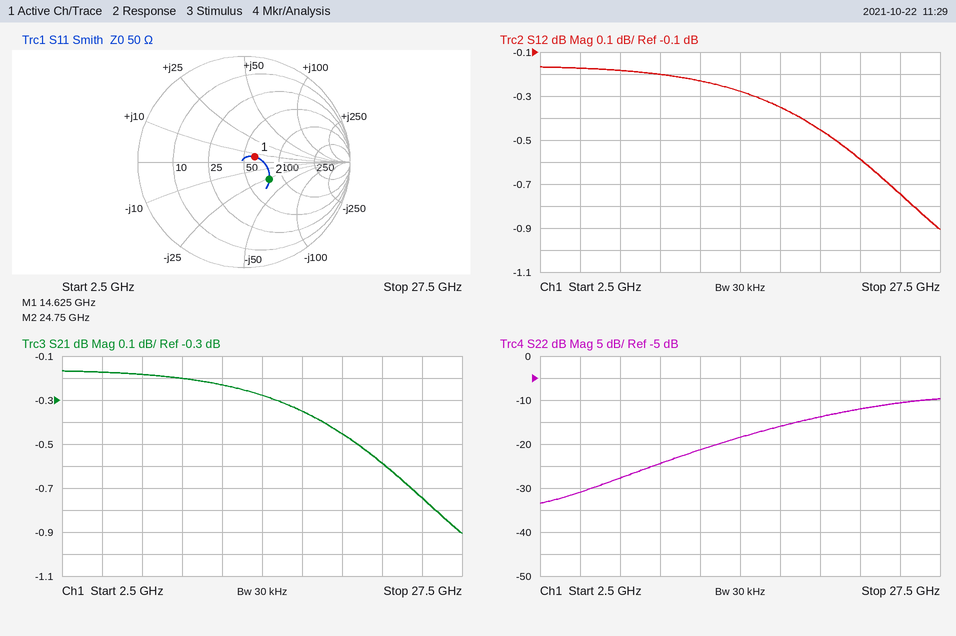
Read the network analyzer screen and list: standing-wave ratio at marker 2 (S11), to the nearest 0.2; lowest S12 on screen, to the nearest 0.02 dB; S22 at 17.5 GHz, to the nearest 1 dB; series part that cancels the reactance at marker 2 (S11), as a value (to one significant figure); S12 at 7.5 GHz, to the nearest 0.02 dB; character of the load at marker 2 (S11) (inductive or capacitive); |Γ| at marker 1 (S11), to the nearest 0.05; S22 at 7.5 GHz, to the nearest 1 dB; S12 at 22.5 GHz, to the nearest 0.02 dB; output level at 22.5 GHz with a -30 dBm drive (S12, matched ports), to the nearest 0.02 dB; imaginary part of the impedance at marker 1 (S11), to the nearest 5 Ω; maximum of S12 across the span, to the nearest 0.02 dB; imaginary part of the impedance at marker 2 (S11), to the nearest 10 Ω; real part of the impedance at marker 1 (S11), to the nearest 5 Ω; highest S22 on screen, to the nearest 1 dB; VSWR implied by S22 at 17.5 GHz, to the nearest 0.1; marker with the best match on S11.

1.8
-0.90 dB
-16 dB
200 pH
-0.18 dB
capacitive
0.10
-28 dB
-0.58 dB
-30.58 dBm
+5 Ω
-0.16 dB
-30 Ω
60 Ω
-10 dB
1.4
marker 1
